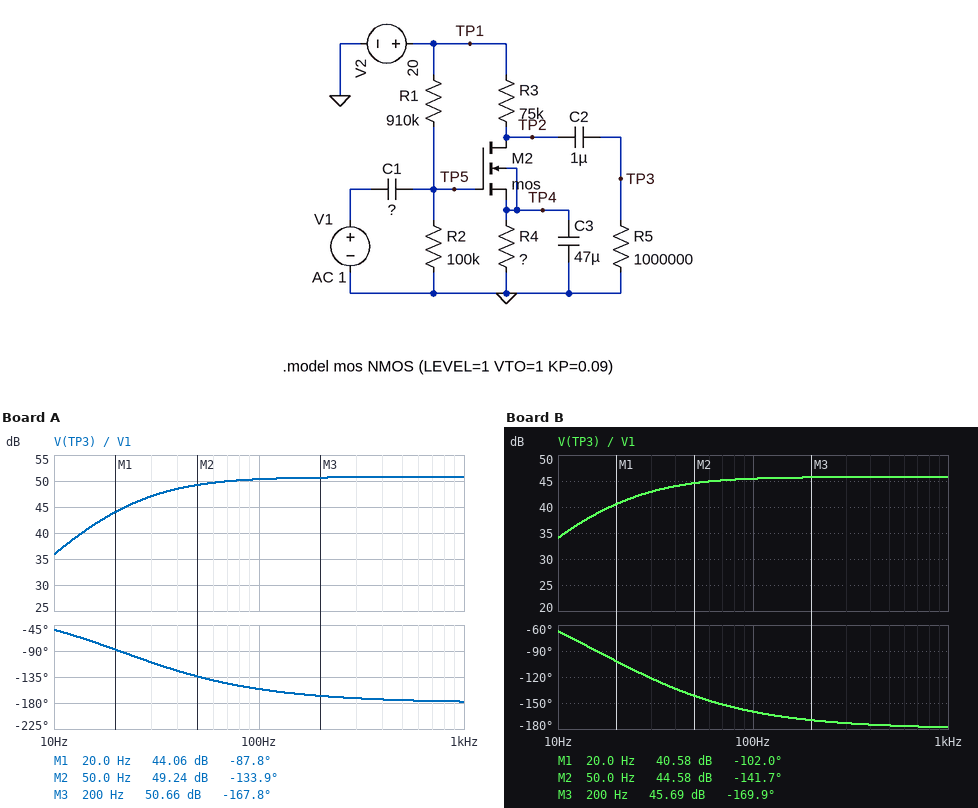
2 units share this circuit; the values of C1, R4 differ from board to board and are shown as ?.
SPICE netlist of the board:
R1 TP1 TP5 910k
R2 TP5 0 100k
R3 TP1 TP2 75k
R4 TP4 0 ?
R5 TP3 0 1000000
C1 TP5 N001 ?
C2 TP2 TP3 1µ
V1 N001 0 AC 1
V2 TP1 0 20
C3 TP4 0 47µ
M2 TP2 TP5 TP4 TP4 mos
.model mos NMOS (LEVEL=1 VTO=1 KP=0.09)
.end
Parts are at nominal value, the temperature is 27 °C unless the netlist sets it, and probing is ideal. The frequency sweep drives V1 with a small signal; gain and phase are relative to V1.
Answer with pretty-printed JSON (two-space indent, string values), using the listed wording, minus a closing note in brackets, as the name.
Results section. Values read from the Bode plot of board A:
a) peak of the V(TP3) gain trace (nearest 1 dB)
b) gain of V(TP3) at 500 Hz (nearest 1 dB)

{
  "peak of the V(TP3) gain trace": "51 dB",
  "gain of V(TP3) at 500 Hz": "51 dB"
}
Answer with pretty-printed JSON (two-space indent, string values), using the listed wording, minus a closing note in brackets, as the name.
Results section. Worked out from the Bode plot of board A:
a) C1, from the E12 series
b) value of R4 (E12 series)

{
  "C1, from the E12 series": "68 nF",
  "value of R4": "6.8 kΩ"
}
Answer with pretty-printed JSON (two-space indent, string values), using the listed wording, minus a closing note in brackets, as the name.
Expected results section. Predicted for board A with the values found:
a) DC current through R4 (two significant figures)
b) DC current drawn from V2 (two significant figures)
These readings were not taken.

{
  "DC current through R4": "140 µA",
  "DC current drawn from V2": "160 µA"
}
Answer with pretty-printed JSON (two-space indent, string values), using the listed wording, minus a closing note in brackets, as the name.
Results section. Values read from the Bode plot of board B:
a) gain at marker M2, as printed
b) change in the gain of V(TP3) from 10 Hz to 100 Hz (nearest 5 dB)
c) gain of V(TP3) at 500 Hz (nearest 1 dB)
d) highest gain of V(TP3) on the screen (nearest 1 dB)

{
  "gain at marker M2, as printed": "44.58 dB",
  "change in the gain of V(TP3) from 10 Hz to 100 Hz": "10 dB",
  "gain of V(TP3) at 500 Hz": "46 dB",
  "highest gain of V(TP3) on the screen": "46 dB"
}
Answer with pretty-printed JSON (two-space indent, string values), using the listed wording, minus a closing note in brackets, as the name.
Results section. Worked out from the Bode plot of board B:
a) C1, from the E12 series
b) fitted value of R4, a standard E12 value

{
  "C1, from the E12 series": "68 nF",
  "fitted value of R4, a standard E12 value": "22 kΩ"
}
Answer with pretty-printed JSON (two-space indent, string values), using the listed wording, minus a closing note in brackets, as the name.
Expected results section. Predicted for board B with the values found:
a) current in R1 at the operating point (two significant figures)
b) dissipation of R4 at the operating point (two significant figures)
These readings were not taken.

{
  "current in R1 at the operating point": "20 µA",
  "dissipation of R4 at the operating point": "41 µW"
}
